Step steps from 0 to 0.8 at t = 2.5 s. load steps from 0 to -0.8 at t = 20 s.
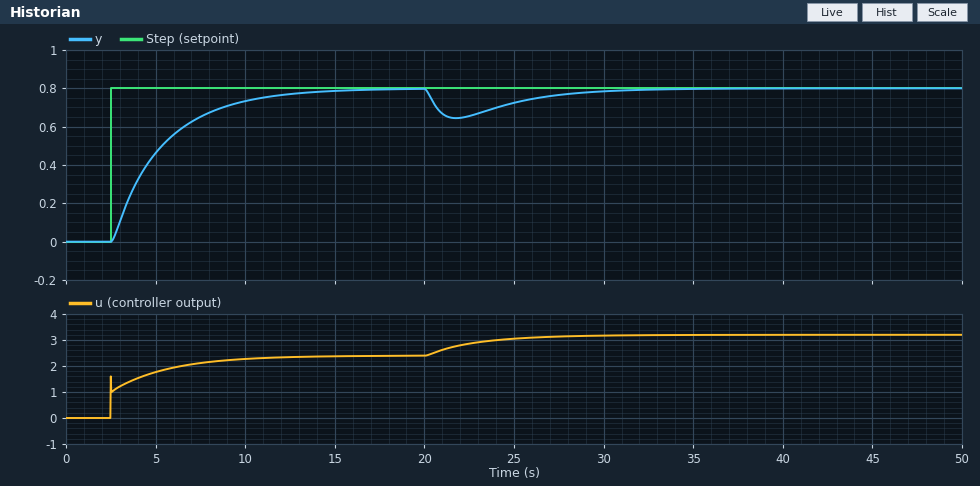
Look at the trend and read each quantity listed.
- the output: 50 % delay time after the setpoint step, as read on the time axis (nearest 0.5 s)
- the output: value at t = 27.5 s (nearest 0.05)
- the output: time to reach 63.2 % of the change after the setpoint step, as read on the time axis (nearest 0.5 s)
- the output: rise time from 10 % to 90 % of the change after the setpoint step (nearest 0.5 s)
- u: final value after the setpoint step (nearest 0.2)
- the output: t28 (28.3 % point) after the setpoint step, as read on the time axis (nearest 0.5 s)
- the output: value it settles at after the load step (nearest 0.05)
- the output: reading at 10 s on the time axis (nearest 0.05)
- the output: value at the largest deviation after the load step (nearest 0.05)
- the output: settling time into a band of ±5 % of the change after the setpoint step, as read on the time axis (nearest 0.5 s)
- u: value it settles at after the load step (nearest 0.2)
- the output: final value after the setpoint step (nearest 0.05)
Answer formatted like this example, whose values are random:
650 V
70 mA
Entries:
4.5 s
0.75
5.5 s
6.5 s
2.4
3.5 s
0.80
0.75
0.65
11.5 s
3.2
0.80
